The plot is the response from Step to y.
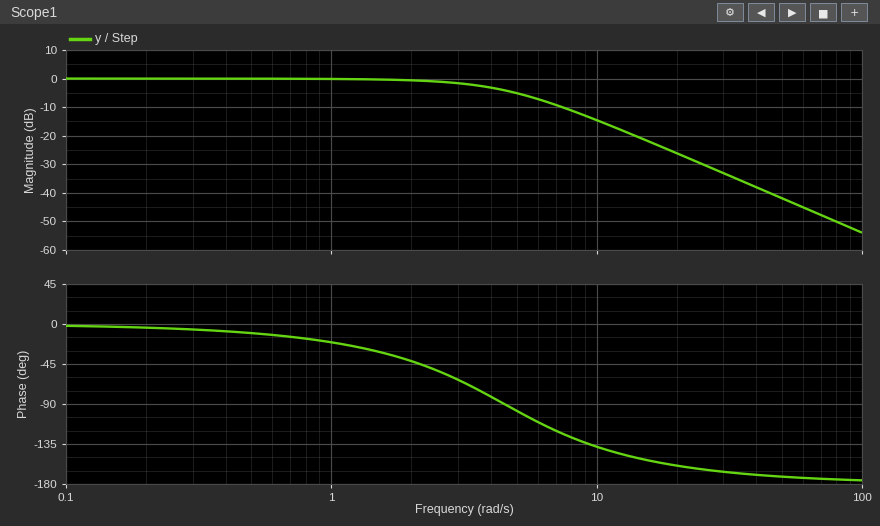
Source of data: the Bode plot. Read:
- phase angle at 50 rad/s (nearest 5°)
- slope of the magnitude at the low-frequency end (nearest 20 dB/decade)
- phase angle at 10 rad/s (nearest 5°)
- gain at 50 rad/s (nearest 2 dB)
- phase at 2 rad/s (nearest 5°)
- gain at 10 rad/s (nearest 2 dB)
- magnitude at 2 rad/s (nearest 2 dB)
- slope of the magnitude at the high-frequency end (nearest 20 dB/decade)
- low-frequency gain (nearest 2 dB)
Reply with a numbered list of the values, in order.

1. -170°
2. 0 dB/decade
3. -140°
4. -42 dB
5. -40°
6. -14 dB
7. 0 dB
8. -40 dB/decade
9. 0 dB
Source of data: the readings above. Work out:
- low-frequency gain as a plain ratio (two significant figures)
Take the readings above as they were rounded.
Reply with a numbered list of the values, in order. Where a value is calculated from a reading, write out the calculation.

1. 10^(0 / 20) = 1.0
